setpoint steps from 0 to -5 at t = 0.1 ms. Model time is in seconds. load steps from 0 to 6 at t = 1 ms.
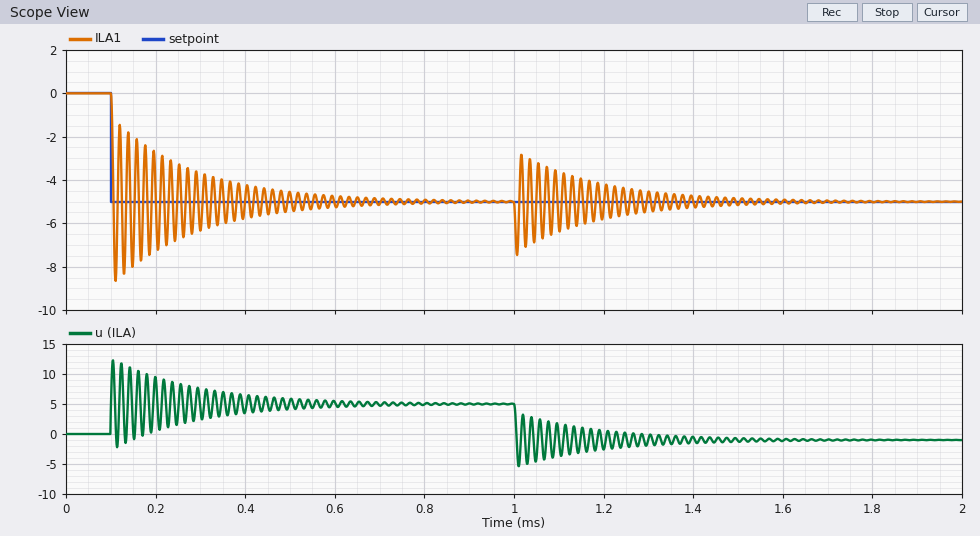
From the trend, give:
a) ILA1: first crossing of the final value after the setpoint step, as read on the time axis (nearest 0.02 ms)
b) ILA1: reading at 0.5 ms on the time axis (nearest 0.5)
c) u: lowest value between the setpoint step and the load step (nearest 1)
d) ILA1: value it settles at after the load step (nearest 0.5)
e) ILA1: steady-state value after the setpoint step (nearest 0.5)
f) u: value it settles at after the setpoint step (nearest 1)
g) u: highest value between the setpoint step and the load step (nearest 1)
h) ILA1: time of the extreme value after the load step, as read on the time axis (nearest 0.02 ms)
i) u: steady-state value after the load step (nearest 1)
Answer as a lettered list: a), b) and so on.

a) 0.10 ms
b) -4.5
c) -2
d) -5.0
e) -5.0
f) 5
g) 12
h) 1.00 ms
i) -1
